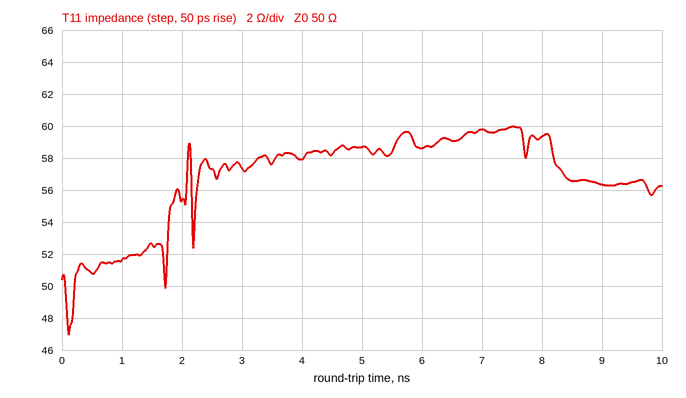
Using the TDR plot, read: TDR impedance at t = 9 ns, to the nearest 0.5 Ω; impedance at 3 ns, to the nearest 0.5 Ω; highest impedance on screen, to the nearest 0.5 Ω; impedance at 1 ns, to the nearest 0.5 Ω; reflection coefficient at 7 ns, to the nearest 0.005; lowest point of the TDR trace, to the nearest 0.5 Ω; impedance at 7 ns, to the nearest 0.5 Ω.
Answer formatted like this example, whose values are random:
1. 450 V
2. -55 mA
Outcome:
1. 56.5 Ω
2. 57.5 Ω
3. 60.0 Ω
4. 51.5 Ω
5. +0.090
6. 47.0 Ω
7. 60.0 Ω
